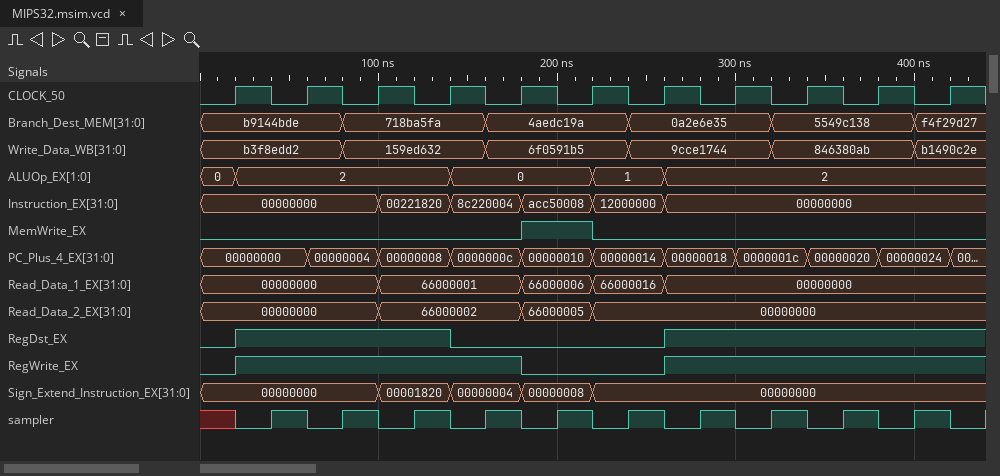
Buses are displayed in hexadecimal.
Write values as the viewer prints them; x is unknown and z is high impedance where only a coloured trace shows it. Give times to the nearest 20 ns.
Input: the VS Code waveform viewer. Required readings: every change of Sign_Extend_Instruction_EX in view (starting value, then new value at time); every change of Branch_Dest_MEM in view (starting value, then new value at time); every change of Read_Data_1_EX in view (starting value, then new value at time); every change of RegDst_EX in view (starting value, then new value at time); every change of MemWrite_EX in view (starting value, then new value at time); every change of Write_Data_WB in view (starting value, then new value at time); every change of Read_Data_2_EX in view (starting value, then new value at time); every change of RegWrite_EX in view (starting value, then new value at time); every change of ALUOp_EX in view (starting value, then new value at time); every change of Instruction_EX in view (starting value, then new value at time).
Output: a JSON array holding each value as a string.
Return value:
["00000000, 00001820 at 100 ns, 00000004 at 140 ns, 00000008 at 180 ns, 00000000 at 220 ns", "b9144bde, 718ba5fa at 80 ns, 4aedc19a at 160 ns, 0a2e6e35 at 240 ns, 5549c138 at 320 ns, f4f29d27 at 400 ns", "00000000, 66000001 at 100 ns, 66000006 at 180 ns, 66000016 at 220 ns, 00000000 at 260 ns", "0, 1 at 20 ns, 0 at 140 ns, 1 at 260 ns", "0, 1 at 180 ns, 0 at 220 ns", "b3f8edd2, 159ed632 at 80 ns, 6f0591b5 at 160 ns, 9cce1744 at 240 ns, 846380ab at 320 ns, b1490c2e at 400 ns", "00000000, 66000002 at 100 ns, 66000005 at 180 ns, 00000000 at 220 ns", "0, 1 at 20 ns, 0 at 180 ns, 1 at 260 ns", "0, 2 at 20 ns, 0 at 140 ns, 1 at 220 ns, 2 at 260 ns", "00000000, 00221820 at 100 ns, 8c220004 at 140 ns, acc50008 at 180 ns, 12000000 at 220 ns, 00000000 at 260 ns"]
